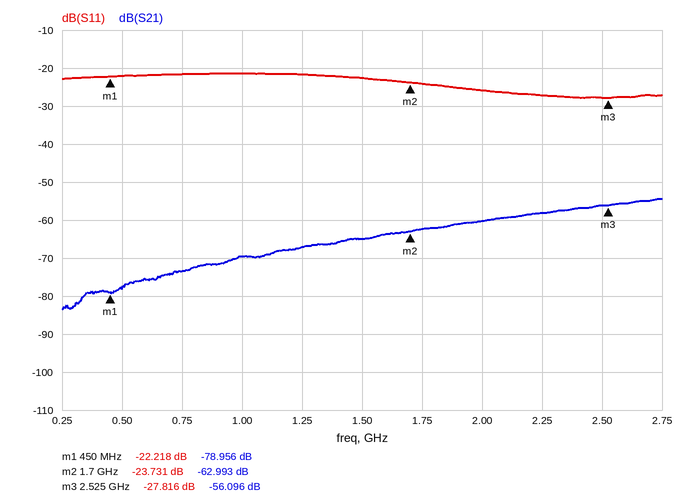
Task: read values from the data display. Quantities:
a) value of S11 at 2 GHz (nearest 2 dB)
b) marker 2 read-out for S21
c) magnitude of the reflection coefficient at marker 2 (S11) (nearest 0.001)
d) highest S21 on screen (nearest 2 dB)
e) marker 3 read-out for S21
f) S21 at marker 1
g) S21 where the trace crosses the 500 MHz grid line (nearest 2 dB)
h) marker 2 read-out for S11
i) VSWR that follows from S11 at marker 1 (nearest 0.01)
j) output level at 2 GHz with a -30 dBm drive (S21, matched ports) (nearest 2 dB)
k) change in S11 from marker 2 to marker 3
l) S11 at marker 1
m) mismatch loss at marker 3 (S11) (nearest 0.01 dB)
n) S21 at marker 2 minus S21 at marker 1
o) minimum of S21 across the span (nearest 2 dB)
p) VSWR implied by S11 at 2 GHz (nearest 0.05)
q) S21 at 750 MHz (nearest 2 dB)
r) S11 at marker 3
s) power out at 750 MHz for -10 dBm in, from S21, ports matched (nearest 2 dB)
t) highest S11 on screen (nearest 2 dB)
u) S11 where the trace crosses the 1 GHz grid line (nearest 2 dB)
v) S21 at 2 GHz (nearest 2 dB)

-26 dB
-62.993 dB
0.065
-54 dB
-56.096 dB
-78.956 dB
-78 dB
-23.731 dB
1.17
-90 dBm
-4.085 dB
-22.218 dB
0.01 dB
15.963 dB
-84 dB
1.10
-74 dB
-27.816 dB
-84 dBm
-22 dB
-22 dB
-60 dB
